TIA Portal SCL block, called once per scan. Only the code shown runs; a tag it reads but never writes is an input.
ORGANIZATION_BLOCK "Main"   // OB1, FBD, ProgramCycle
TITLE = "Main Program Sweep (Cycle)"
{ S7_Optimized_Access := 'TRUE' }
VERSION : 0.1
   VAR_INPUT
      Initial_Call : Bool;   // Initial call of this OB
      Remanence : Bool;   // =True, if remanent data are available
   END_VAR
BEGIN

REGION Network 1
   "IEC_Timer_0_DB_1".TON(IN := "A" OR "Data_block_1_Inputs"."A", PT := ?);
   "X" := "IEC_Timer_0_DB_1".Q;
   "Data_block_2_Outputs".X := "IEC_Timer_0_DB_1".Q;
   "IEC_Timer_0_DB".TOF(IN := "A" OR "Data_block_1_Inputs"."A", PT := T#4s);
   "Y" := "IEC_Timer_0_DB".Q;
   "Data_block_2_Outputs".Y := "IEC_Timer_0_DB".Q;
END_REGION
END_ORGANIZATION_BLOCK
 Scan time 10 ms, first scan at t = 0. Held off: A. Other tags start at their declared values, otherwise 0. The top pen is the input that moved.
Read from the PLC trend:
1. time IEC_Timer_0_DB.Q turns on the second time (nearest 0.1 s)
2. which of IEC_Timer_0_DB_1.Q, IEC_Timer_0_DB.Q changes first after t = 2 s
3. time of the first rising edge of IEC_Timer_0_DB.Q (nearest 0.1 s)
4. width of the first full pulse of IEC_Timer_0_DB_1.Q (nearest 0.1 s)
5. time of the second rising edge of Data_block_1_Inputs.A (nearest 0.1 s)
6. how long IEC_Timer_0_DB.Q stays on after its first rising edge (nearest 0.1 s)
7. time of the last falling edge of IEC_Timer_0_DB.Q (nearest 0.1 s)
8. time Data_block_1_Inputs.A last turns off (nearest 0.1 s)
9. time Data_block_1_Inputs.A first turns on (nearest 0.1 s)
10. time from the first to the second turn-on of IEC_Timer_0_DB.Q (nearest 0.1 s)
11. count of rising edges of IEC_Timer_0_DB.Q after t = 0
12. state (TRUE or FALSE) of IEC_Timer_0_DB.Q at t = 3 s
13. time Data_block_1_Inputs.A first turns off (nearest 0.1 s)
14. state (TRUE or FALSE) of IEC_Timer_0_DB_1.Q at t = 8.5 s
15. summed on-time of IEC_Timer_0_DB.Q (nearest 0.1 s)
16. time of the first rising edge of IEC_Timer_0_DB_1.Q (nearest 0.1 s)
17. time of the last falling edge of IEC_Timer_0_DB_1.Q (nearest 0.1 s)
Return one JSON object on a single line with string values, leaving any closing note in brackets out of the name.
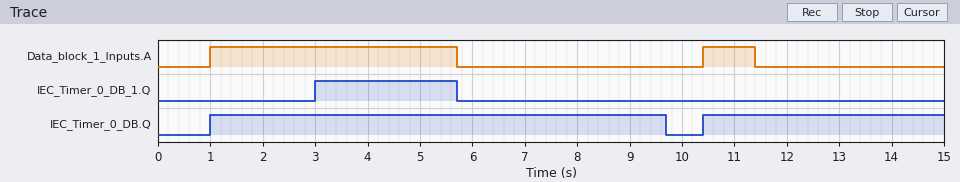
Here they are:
{"time IEC_Timer_0_DB.Q turns on the second time": "10.4 s", "which of IEC_Timer_0_DB_1.Q, IEC_Timer_0_DB.Q changes first after t = 2 s": "IEC_Timer_0_DB_1.Q", "time of the first rising edge of IEC_Timer_0_DB.Q": "1.0 s", "width of the first full pulse of IEC_Timer_0_DB_1.Q": "2.7 s", "time of the second rising edge of Data_block_1_Inputs.A": "10.4 s", "how long IEC_Timer_0_DB.Q stays on after its first rising edge": "8.7 s", "time of the last falling edge of IEC_Timer_0_DB.Q": "9.7 s", "time Data_block_1_Inputs.A last turns off": "11.4 s", "time Data_block_1_Inputs.A first turns on": "1.0 s", "time from the first to the second turn-on of IEC_Timer_0_DB.Q": "9.4 s", "count of rising edges of IEC_Timer_0_DB.Q after t = 0": "2", "state (TRUE or FALSE) of IEC_Timer_0_DB.Q at t = 3 s": "TRUE", "time Data_block_1_Inputs.A first turns off": "5.7 s", "state (TRUE or FALSE) of IEC_Timer_0_DB_1.Q at t = 8.5 s": "FALSE", "summed on-time of IEC_Timer_0_DB.Q": "13.3 s", "time of the first rising edge of IEC_Timer_0_DB_1.Q": "3.0 s", "time of the last falling edge of IEC_Timer_0_DB_1.Q": "5.7 s"}
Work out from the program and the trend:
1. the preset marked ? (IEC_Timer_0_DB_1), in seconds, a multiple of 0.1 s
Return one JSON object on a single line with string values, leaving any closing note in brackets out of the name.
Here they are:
{"the preset marked ? (IEC_Timer_0_DB_1), in seconds, a multiple of 0.1 s": "2.0 s"}
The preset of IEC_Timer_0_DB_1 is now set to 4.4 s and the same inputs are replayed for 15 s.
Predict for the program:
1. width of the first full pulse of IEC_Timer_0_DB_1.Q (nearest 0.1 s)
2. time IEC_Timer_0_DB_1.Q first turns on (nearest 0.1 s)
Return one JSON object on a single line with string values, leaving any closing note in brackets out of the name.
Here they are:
{"width of the first full pulse of IEC_Timer_0_DB_1.Q": "0.3 s", "time IEC_Timer_0_DB_1.Q first turns on": "5.4 s"}
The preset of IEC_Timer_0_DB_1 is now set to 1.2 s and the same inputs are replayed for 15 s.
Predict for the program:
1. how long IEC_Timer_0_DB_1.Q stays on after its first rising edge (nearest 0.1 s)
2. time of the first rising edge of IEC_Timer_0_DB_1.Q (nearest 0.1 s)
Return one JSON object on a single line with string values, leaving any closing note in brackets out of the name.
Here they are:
{"how long IEC_Timer_0_DB_1.Q stays on after its first rising edge": "3.5 s", "time of the first rising edge of IEC_Timer_0_DB_1.Q": "2.2 s"}
